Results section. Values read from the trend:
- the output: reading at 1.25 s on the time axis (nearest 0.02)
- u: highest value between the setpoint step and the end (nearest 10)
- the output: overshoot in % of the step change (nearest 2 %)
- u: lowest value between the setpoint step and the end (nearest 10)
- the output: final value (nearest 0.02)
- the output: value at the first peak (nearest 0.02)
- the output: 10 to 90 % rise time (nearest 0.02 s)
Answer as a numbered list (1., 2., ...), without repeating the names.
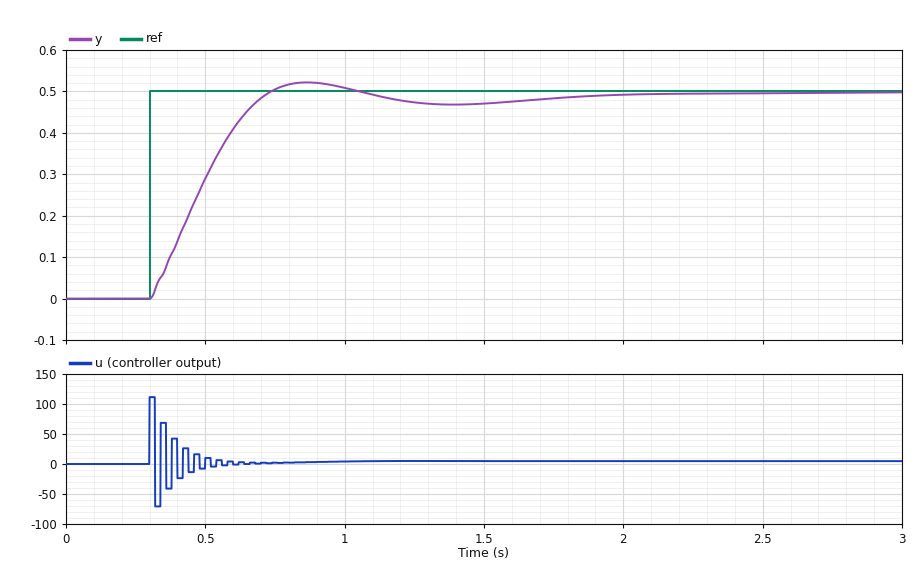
1. 0.48
2. 110
3. 4 %
4. -70
5. 0.50
6. 0.52
7. 0.30 s
